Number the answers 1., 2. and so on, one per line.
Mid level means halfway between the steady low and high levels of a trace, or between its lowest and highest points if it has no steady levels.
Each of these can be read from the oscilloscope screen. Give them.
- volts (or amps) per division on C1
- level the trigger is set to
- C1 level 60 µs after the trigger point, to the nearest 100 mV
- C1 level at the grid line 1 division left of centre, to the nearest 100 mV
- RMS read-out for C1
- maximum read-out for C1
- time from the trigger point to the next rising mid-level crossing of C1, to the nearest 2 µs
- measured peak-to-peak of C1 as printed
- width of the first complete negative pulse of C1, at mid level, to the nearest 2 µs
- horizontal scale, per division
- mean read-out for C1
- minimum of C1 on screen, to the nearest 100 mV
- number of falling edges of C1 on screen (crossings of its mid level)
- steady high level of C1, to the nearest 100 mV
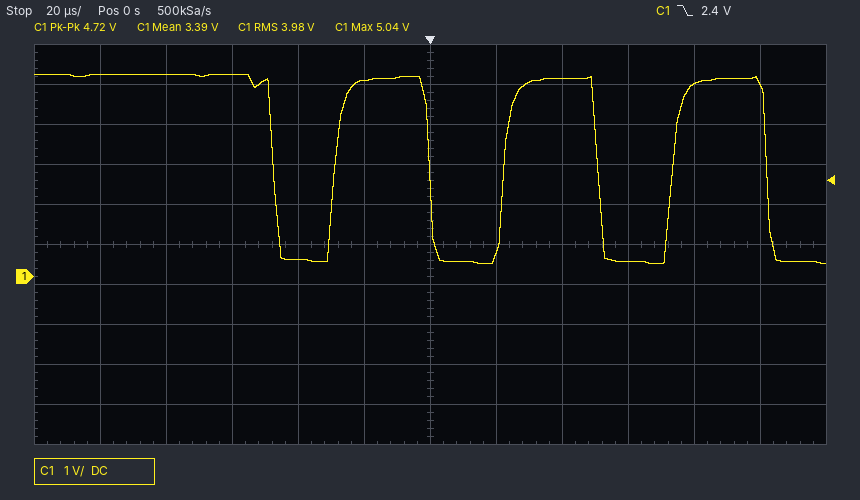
1. 1 V
2. 2.4 V
3. 400 mV
4. 4.9 V
5. 3.98 V
6. 5.04 V
7. 22 µs
8. 4.72 V
9. 18 µs
10. 20 µs
11. 3.39 V
12. 300 mV
13. 4
14. 5.0 V
